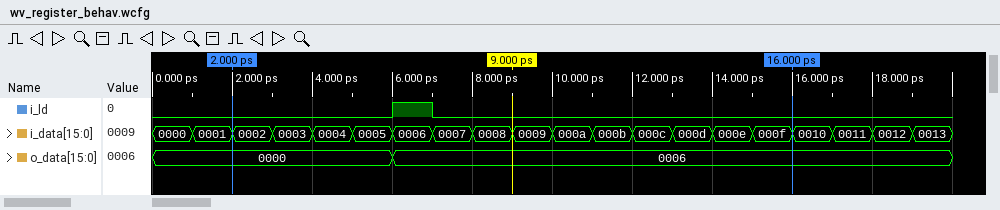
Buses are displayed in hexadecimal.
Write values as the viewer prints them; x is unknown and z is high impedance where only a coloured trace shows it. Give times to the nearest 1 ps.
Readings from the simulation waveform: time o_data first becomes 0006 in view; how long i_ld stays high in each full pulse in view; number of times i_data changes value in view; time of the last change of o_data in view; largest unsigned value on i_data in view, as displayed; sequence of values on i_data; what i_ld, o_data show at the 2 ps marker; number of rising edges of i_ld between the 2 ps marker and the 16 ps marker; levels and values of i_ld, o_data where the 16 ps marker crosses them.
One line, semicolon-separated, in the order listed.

6 ps; 1 ps; 19; 6 ps; 0013; 0000, 0001, 0002, 0003, 0004, 0005, 0006, 0007, 0008, 0009, 000a, 000b, 000c, 000d, 000e, 000f, 0010, 0011, 0012, 0013; i_ld=0, o_data=0000; 1; i_ld=0, o_data=0006
